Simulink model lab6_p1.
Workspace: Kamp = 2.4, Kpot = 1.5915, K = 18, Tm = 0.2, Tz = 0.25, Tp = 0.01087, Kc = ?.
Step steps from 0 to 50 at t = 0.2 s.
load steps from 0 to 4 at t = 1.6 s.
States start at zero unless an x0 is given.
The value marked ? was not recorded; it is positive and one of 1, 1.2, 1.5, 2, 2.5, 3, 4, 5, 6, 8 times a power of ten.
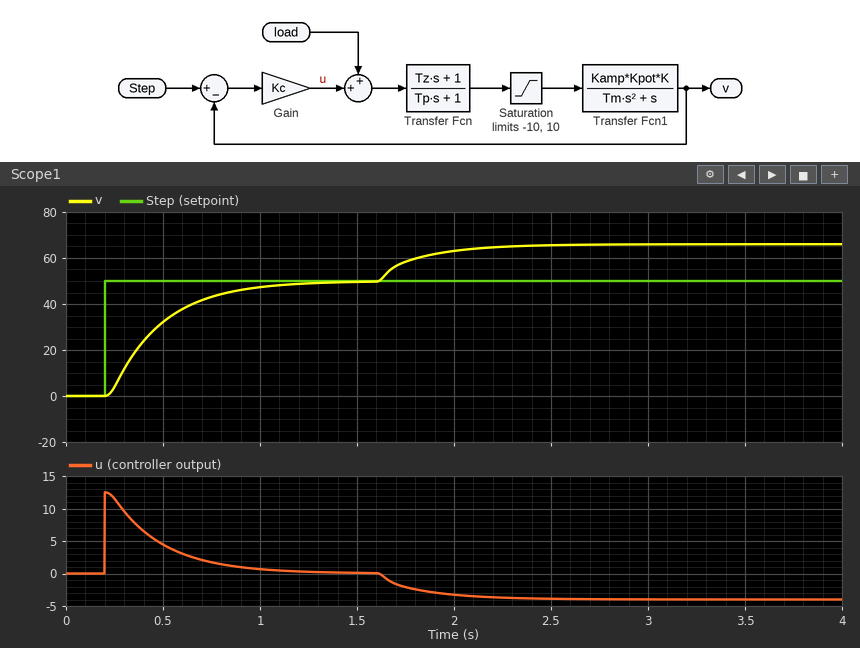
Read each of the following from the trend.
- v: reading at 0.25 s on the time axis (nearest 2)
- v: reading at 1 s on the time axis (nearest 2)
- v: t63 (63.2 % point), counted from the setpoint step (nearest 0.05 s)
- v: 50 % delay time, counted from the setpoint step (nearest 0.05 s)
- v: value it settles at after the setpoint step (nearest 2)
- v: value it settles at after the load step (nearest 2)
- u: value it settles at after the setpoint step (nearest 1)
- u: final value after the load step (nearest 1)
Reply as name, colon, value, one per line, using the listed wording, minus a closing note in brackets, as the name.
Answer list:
v: reading at 0.25 s on the time axis: 4
v: reading at 1 s on the time axis: 48
v: t63 (63.2 % point), counted from the setpoint step: 0.30 s
v: 50 % delay time, counted from the setpoint step: 0.20 s
v: value it settles at after the setpoint step: 50
v: value it settles at after the load step: 66
u: value it settles at after the setpoint step: 0
u: final value after the load step: -4
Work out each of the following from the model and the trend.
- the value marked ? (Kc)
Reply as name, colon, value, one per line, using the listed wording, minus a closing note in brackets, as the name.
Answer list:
the value marked ?: 0.25
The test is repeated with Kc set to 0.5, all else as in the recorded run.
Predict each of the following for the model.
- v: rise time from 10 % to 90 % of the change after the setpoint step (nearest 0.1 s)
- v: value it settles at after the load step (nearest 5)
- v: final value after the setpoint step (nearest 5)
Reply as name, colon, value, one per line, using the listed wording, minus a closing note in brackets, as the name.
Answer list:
v: rise time from 10 % to 90 % of the change after the setpoint step: 0.6 s
v: value it settles at after the load step: 60
v: final value after the setpoint step: 50
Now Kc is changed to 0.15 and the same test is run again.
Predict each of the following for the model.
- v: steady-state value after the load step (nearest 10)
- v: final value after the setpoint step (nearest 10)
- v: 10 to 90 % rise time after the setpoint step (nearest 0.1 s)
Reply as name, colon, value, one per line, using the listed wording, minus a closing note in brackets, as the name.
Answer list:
v: steady-state value after the load step: 80
v: final value after the setpoint step: 50
v: 10 to 90 % rise time after the setpoint step: 0.6 s
